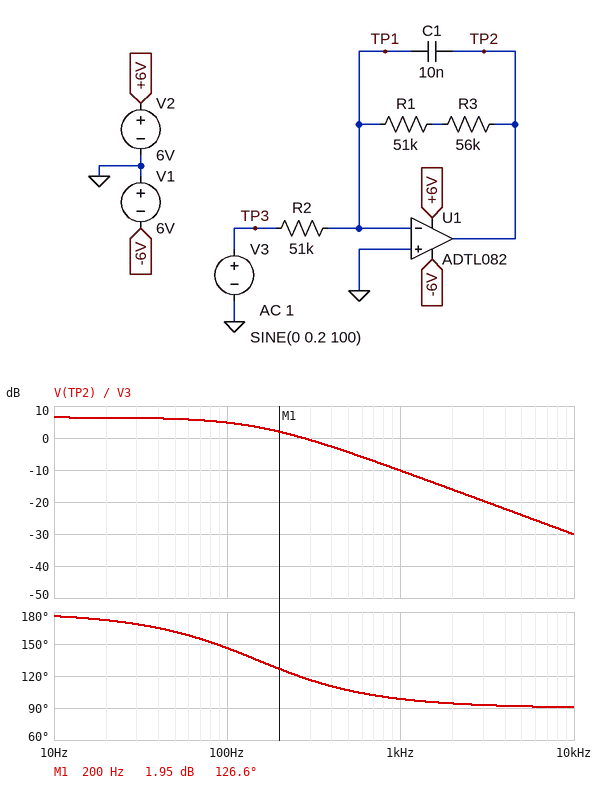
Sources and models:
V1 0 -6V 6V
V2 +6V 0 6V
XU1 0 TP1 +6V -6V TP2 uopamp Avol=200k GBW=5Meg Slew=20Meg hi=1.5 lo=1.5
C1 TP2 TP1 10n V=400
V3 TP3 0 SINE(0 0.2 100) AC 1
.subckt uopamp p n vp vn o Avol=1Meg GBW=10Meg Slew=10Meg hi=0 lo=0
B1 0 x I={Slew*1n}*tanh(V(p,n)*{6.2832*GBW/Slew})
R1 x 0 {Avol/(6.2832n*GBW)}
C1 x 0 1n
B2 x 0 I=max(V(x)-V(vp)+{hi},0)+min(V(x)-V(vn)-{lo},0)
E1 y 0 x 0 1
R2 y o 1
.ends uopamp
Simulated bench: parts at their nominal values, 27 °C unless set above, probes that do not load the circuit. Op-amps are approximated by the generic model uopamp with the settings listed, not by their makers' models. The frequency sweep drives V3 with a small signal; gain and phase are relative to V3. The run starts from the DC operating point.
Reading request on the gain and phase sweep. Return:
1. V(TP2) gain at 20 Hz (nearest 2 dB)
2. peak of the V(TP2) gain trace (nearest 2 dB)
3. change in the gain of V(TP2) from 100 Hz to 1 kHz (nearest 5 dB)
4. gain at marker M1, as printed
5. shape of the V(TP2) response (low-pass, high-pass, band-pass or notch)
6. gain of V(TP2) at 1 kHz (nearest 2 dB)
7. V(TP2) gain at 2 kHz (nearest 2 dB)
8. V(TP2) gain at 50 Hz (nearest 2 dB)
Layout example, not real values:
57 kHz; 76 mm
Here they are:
6 dB; 6 dB; -15 dB; 1.95 dB; low-pass; -10 dB; -16 dB; 6 dB
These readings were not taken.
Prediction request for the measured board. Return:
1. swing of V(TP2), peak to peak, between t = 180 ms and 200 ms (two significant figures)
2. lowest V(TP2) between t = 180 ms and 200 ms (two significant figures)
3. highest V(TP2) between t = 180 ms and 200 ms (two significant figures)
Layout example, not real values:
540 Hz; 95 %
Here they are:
700 mV; -350 mV; 350 mV
